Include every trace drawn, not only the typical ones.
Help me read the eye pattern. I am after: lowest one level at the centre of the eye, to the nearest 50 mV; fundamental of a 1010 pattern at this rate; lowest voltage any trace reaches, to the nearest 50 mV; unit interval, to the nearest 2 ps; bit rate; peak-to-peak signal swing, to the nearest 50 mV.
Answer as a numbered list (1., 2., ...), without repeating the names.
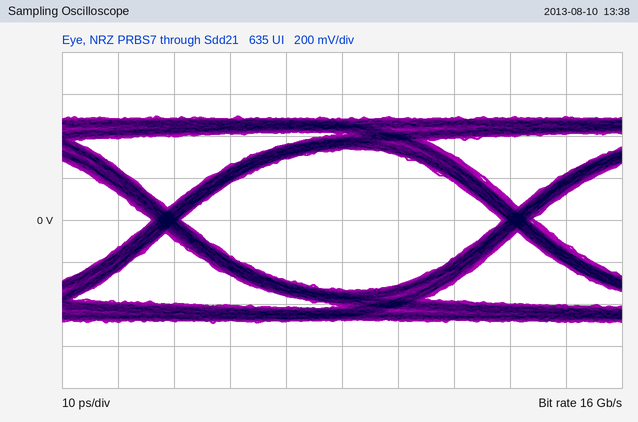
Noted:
1. 350 mV
2. 8 GHz
3. -500 mV
4. 62 ps
5. 16 Gb/s
6. 1.00 V
